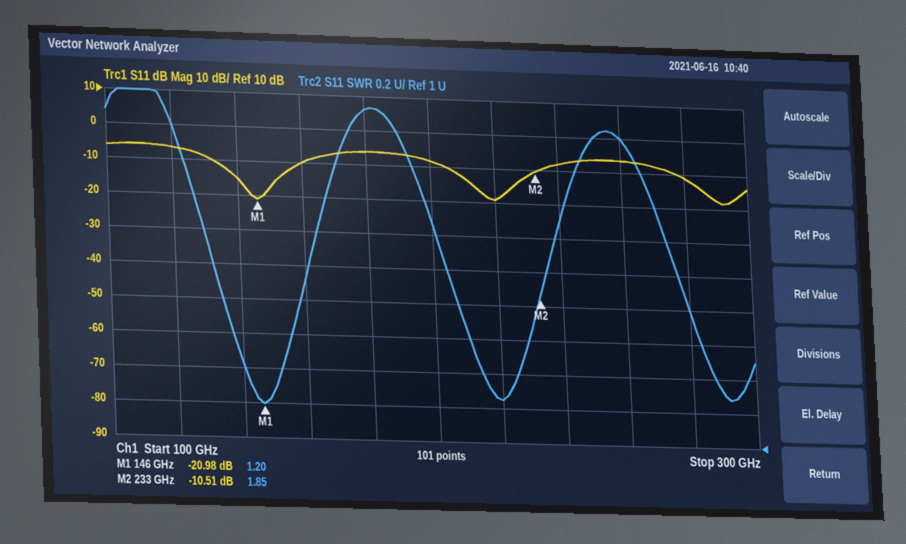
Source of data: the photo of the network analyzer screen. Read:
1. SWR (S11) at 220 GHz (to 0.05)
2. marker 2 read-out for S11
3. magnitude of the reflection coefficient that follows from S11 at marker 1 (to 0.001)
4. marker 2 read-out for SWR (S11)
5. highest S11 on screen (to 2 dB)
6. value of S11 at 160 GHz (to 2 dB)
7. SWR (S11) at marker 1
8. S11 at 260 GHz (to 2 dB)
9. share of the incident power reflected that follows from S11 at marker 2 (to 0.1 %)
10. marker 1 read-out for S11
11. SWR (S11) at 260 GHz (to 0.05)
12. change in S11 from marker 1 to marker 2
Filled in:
1.25
-10.51 dB
0.089
1.85
-6 dB
-10 dB
1.20
-6 dB
8.9 %
-20.98 dB
2.80
10.47 dB
